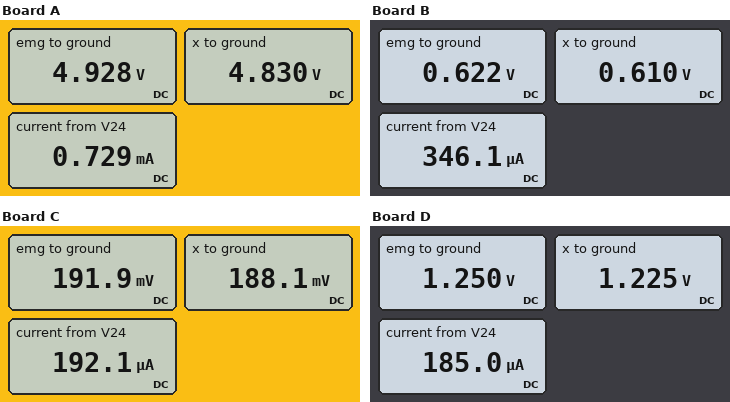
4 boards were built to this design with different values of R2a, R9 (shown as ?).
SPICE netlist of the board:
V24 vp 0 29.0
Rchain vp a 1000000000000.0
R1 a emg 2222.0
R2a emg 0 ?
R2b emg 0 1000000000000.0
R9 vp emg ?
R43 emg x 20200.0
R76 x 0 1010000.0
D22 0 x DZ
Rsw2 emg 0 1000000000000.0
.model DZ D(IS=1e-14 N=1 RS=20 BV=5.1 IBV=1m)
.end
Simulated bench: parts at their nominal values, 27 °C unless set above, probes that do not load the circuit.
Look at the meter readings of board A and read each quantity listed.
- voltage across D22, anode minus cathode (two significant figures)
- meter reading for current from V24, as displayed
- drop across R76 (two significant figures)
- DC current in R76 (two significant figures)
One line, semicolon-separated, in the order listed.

-4.8 V; 0.729 mA; 4.8 V; 4.8 µA
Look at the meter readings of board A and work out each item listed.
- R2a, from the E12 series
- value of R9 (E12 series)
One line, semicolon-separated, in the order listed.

6.8 kΩ; 33 kΩ
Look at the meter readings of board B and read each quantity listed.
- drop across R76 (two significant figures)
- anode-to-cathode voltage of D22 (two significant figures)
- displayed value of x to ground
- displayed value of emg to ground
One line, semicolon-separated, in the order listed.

610 mV; -610 mV; 0.610 V; 0.622 V
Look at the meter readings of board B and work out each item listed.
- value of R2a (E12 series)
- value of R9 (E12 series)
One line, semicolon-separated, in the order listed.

1.8 kΩ; 82 kΩ
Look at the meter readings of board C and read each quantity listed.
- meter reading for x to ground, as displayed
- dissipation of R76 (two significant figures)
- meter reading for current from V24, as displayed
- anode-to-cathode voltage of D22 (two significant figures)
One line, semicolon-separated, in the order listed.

188.1 mV; 35 nW; 192.1 µA; -190 mV
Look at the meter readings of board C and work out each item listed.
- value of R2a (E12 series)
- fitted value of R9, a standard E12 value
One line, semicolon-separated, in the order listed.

1 kΩ; 150 kΩ
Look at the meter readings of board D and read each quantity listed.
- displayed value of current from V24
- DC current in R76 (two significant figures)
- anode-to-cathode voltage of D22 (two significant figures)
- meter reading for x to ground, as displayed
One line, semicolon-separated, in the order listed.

185.0 µA; 1.2 µA; -1.2 V; 1.225 V
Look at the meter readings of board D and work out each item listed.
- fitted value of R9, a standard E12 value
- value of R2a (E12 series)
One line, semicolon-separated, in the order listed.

150 kΩ; 6.8 kΩ
